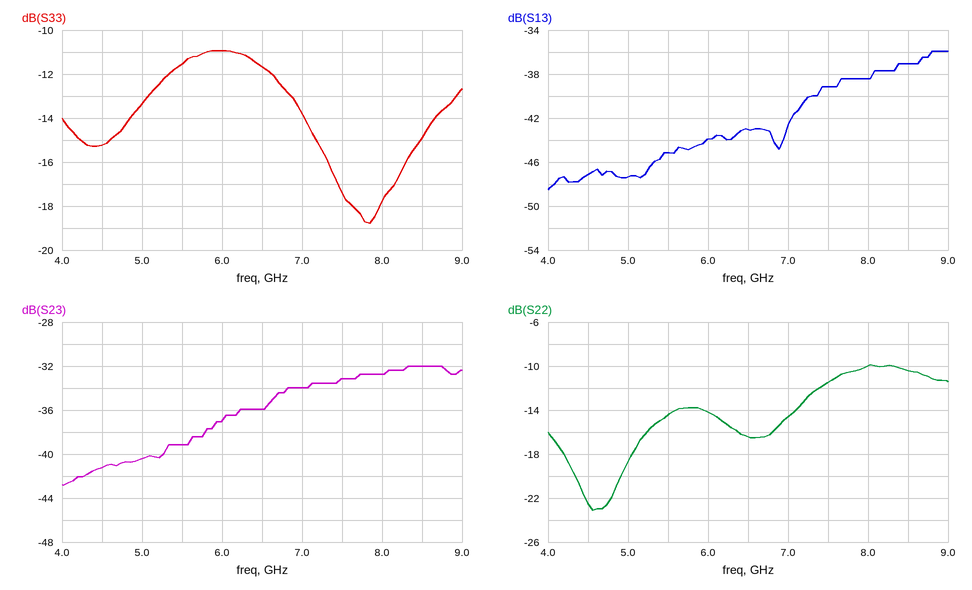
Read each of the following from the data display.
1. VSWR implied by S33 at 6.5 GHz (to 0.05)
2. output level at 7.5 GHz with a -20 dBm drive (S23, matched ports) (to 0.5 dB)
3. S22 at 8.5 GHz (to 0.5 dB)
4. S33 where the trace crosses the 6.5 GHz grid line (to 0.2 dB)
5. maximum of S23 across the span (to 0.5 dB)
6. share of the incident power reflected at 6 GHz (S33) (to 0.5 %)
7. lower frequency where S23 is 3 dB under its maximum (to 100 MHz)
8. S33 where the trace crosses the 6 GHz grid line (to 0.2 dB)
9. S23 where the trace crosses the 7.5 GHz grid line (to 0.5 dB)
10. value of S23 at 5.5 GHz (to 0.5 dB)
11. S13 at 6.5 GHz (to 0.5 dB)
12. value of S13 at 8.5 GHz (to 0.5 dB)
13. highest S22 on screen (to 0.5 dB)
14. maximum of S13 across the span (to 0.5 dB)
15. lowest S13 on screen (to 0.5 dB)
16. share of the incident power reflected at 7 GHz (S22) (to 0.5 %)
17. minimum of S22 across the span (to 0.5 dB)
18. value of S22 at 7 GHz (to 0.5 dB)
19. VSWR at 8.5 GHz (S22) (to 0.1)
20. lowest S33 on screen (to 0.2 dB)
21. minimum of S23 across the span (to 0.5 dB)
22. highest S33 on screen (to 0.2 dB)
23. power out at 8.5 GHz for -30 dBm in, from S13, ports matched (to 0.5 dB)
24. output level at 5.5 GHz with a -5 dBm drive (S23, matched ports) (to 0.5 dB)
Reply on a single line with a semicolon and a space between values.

1.70; -53.0 dBm; -10.5 dB; -11.6 dB; -32.0 dB; 8.0 %; 6.6 GHz; -11.0 dB; -33.0 dB; -39.0 dB; -43.0 dB; -37.0 dB; -10.0 dB; -36.0 dB; -48.5 dB; 3.5 %; -23.0 dB; -14.5 dB; 1.9; -18.8 dB; -43.0 dB; -11.0 dB; -67.0 dBm; -44.0 dBm
